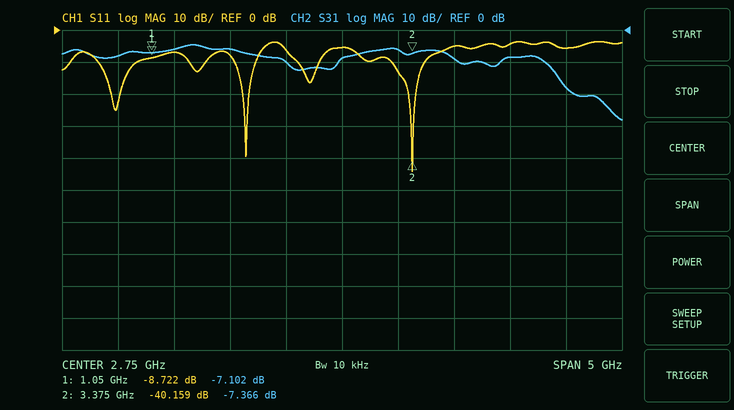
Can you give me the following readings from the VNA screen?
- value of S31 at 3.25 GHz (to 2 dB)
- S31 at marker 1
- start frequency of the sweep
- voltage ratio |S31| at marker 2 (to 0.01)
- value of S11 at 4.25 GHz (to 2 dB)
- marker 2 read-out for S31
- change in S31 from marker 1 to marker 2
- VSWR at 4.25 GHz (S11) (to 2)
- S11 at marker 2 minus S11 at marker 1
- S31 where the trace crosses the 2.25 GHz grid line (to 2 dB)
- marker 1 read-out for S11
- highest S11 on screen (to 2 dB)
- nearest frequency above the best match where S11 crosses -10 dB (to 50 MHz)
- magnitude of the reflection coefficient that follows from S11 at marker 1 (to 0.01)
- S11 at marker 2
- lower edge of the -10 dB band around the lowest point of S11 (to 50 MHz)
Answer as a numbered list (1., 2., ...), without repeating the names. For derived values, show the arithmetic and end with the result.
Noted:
1. -6 dB
2. -7.102 dB
3. 250 MHz
4. 10^(-7.366/20) ≈ 0.43
5. -4 dB
6. -7.366 dB
7. -7.366 − (-7.102) = -0.264 dB
8. |Γ| = 10^(-4/20) = 0.6310; VSWR = (1 + 0.6310)/(1 − 0.6310) ≈ 4
9. -40.159 − (-8.722) = -31.437 dB
10. -10 dB
11. -8.722 dB
12. -4 dB
13. 3.50 GHz
14. 10^(-8.722/20) ≈ 0.37
15. -40.159 dB
16. 3.20 GHz
